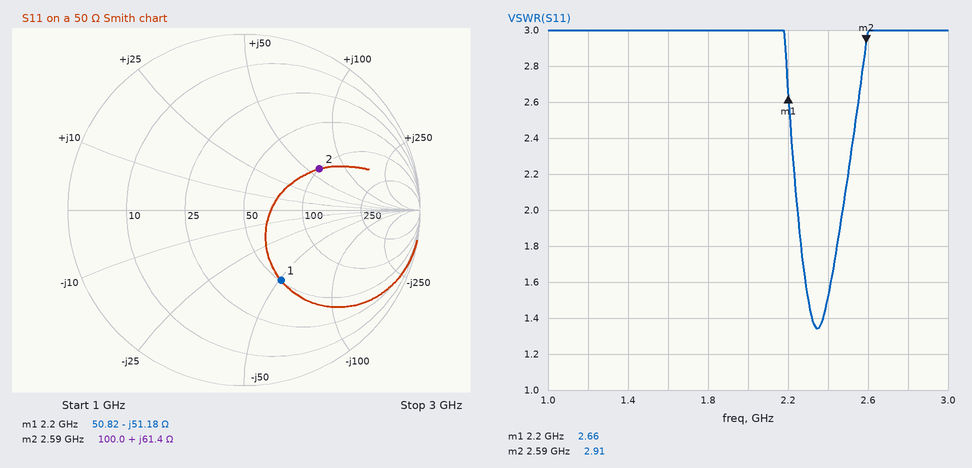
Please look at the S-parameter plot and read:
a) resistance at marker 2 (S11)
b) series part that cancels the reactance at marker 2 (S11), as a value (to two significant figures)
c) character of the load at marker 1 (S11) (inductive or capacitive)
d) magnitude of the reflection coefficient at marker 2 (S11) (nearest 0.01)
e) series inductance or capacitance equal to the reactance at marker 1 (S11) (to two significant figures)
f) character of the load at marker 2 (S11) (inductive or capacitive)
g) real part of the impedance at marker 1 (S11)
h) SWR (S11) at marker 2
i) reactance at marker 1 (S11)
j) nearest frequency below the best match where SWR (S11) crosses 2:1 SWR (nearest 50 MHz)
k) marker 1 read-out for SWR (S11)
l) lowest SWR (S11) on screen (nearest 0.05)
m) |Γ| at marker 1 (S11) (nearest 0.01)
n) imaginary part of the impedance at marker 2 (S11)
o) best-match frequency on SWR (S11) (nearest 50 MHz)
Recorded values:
100.0 Ω
1.0 pF
capacitive
0.49
1.4 pF
inductive
50.82 Ω
2.91
-51.18 Ω
2.25 GHz
2.66
1.35
0.45
+61.4 Ω
2.35 GHz
